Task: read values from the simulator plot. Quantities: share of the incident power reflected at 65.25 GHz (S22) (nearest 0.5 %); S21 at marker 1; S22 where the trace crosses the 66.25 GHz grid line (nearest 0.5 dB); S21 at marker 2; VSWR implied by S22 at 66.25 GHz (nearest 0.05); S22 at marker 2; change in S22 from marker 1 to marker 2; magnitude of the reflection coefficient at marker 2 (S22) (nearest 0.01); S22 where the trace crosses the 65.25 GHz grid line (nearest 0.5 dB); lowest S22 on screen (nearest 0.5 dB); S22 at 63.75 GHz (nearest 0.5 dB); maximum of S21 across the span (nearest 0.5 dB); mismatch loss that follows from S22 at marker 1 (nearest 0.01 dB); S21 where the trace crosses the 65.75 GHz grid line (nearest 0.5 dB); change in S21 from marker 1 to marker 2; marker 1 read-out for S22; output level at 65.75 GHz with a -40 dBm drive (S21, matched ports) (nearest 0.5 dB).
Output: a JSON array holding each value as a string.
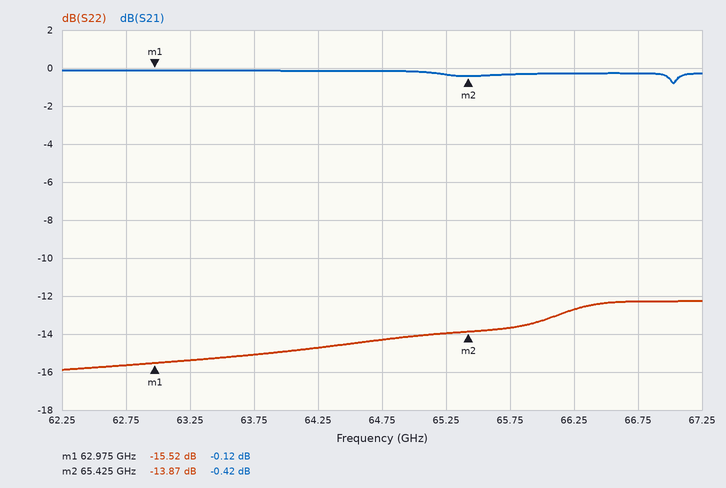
["4.0 %", "-0.12 dB", "-12.5 dB", "-0.42 dB", "1.60", "-13.87 dB", "1.65 dB", "0.20", "-14.0 dB", "-16.0 dB", "-15.0 dB", "0.0 dB", "0.12 dB", "-0.5 dB", "-0.30 dB", "-15.52 dB", "-40.5 dBm"]
